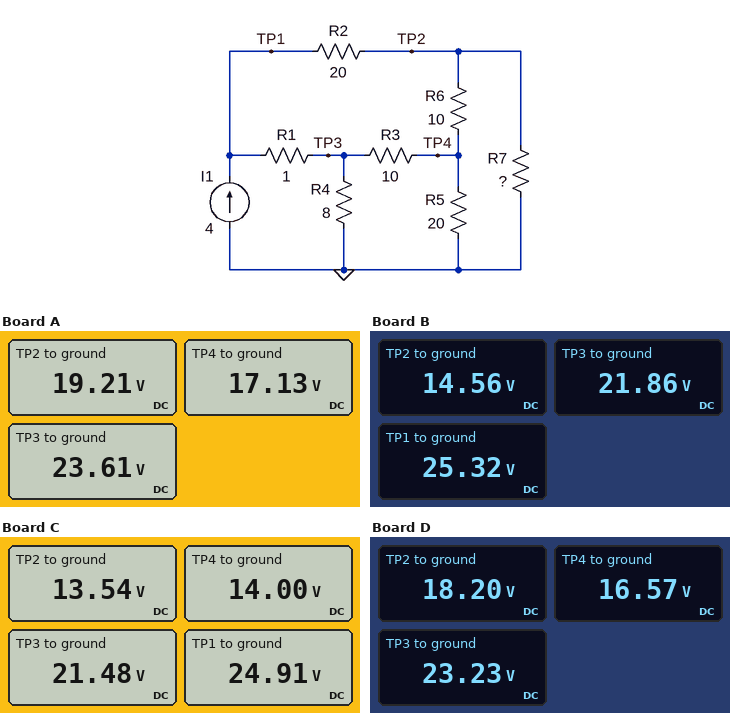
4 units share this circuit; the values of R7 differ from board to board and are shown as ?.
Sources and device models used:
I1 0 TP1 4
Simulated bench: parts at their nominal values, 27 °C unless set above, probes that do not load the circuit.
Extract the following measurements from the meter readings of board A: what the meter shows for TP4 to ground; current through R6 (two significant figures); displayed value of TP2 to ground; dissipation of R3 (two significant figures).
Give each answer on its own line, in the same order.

17.13 V
210 mA
19.21 V
4.2 W
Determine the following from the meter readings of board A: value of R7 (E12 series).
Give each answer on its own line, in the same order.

100 Ω
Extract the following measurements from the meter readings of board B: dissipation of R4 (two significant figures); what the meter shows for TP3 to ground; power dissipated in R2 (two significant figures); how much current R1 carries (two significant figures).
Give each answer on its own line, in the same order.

60 W
21.86 V
5.8 W
3.5 A
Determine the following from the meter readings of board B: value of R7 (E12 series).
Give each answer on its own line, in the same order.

27 Ω
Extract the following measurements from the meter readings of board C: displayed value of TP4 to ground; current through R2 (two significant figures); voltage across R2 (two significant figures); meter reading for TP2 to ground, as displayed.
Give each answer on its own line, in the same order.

14.00 V
570 mA
11 V
13.54 V
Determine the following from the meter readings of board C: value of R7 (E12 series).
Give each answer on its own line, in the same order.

22 Ω
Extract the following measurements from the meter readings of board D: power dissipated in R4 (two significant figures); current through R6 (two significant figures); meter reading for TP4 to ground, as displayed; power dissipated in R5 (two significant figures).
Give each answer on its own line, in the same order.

67 W
160 mA
16.57 V
14 W
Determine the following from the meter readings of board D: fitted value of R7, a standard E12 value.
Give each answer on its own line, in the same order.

68 Ω
